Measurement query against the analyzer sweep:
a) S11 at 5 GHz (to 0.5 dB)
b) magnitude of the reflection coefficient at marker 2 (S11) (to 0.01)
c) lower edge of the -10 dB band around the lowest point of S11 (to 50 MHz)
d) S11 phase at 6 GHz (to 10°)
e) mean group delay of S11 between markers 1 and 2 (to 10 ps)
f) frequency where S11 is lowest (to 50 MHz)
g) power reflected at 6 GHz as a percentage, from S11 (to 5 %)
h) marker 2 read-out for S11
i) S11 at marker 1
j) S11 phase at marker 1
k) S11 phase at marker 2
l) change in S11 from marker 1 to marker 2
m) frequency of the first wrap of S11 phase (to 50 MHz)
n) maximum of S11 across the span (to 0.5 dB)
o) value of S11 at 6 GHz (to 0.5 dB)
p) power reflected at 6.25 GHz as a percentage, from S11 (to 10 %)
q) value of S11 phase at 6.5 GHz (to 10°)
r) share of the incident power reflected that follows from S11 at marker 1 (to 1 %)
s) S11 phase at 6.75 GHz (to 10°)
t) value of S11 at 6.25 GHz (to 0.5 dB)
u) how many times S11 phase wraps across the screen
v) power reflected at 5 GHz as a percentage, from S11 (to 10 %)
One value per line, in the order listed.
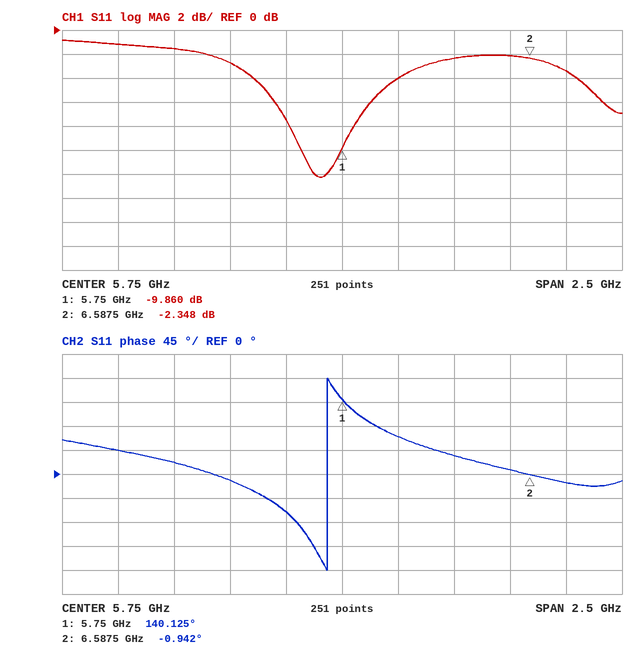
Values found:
-1.5 dB
0.76
5.55 GHz
70°
470 ps
5.65 GHz
40 %
-2.348 dB
-9.860 dB
140.125°
-0.942°
7.512 dB
5.70 GHz
-1.0 dB
-4.0 dB
60 %
10°
10 %
-20°
-2.5 dB
1
70 %
